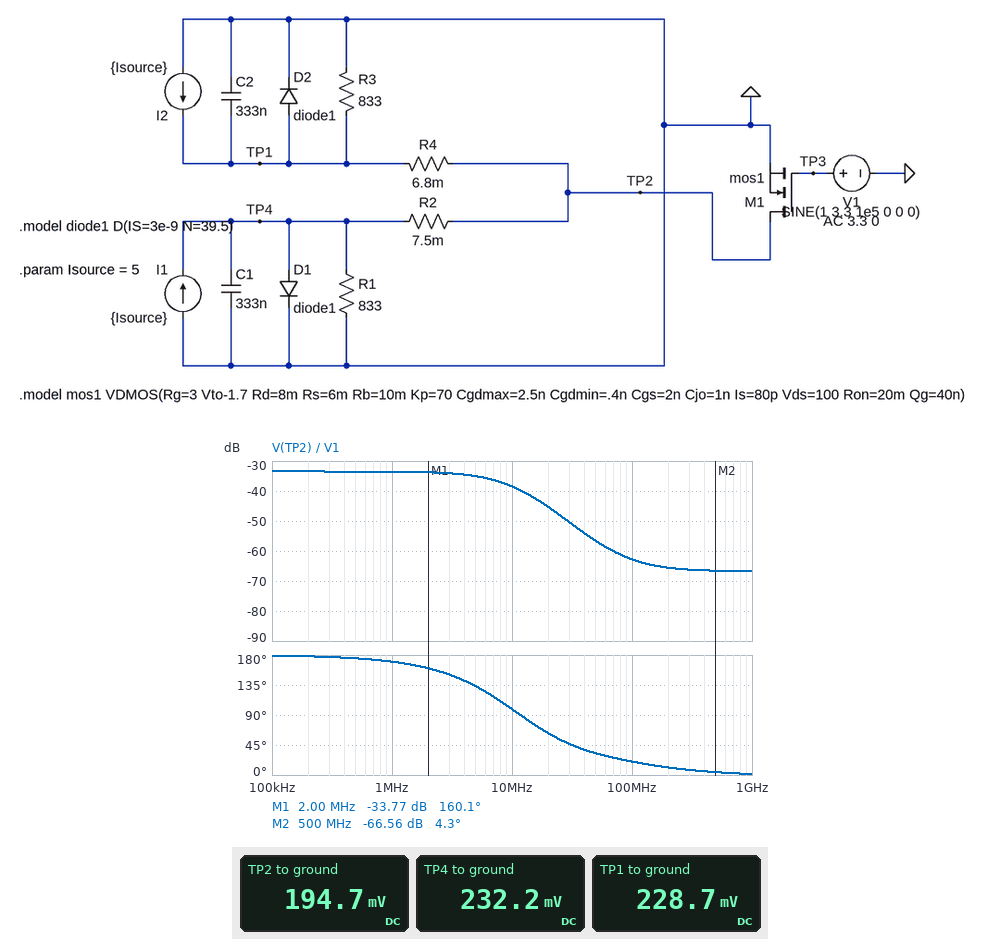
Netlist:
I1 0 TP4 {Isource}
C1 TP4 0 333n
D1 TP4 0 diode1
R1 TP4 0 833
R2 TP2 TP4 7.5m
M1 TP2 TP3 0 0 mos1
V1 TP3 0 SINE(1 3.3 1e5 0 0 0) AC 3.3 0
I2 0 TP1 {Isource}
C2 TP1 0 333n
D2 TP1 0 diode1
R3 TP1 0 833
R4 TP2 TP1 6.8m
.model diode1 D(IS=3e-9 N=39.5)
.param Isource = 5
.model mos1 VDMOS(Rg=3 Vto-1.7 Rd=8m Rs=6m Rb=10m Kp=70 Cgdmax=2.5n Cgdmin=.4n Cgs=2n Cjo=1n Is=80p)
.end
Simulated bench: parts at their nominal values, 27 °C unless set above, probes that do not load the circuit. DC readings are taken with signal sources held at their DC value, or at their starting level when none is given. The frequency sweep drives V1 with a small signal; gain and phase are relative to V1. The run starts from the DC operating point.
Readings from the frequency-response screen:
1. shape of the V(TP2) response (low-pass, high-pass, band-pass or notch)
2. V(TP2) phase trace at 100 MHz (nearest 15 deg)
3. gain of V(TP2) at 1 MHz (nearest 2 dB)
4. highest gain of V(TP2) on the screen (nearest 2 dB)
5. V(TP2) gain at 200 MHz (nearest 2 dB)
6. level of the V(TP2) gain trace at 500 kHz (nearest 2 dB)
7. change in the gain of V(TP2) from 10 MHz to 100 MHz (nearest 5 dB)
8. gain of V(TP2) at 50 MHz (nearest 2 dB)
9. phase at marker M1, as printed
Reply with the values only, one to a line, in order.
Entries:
low-pass
15 deg
-34 dB
-34 dB
-66 dB
-34 dB
-25 dB
-56 dB
160.1 deg
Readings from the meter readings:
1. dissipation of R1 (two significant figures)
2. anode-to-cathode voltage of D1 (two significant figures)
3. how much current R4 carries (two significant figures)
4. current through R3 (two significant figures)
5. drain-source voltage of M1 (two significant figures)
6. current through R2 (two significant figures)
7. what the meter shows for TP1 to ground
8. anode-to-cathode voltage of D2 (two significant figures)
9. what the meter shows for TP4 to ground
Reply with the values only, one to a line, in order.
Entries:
65 µW
230 mV
5.0 A
270 µA
190 mV
5.0 A
228.7 mV
230 mV
232.2 mV
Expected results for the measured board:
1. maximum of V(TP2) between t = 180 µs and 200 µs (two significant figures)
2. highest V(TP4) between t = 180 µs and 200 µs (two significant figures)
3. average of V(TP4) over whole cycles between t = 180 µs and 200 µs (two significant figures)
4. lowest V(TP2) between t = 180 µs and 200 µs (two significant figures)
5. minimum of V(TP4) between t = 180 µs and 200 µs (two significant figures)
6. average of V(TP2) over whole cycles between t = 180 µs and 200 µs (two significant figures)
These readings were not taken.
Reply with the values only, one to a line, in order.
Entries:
22 V
22 V
5.3 V
160 mV
200 mV
5.2 V
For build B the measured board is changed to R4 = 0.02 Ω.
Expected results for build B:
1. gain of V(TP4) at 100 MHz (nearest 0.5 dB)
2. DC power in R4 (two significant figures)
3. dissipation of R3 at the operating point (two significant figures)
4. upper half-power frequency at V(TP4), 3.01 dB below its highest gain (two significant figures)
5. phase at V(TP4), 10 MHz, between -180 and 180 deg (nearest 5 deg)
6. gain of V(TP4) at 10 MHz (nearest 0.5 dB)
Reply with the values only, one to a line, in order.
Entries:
-65.5 dB
500 mW
100 µW
6.9 MHz
95 deg
-39.0 dB
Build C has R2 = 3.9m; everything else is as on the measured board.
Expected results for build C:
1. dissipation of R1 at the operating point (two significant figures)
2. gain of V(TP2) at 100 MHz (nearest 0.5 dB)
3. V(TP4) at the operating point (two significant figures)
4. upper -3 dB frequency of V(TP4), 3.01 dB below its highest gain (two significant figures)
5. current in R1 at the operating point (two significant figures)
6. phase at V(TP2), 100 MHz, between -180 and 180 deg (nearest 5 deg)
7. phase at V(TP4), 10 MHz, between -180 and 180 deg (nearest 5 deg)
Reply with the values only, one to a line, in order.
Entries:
55 µW
-64.0 dB
210 mV
7.4 MHz
260 µA
10 deg
95 deg
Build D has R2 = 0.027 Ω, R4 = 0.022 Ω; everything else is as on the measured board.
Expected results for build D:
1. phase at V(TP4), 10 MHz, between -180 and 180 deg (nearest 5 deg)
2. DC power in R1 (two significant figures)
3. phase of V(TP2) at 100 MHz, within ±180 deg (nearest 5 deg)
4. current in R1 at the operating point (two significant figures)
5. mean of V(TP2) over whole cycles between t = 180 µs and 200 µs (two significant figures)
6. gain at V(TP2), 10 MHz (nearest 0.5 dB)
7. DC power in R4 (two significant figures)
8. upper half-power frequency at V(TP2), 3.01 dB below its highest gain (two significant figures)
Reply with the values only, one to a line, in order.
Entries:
80 deg
130 µW
40 deg
400 µA
5.2 V
-39.0 dB
550 mW
6.5 MHz
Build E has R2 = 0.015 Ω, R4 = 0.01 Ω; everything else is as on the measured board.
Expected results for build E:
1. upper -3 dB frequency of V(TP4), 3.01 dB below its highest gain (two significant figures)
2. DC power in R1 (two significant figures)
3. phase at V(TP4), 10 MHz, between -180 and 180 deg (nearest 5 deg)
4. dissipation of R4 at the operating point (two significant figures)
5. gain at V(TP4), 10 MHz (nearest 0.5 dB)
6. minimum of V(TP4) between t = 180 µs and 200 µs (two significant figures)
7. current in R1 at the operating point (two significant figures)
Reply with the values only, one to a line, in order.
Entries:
6.7 MHz
87 µW
85 deg
250 mW
-39.0 dB
240 mV
320 µA
